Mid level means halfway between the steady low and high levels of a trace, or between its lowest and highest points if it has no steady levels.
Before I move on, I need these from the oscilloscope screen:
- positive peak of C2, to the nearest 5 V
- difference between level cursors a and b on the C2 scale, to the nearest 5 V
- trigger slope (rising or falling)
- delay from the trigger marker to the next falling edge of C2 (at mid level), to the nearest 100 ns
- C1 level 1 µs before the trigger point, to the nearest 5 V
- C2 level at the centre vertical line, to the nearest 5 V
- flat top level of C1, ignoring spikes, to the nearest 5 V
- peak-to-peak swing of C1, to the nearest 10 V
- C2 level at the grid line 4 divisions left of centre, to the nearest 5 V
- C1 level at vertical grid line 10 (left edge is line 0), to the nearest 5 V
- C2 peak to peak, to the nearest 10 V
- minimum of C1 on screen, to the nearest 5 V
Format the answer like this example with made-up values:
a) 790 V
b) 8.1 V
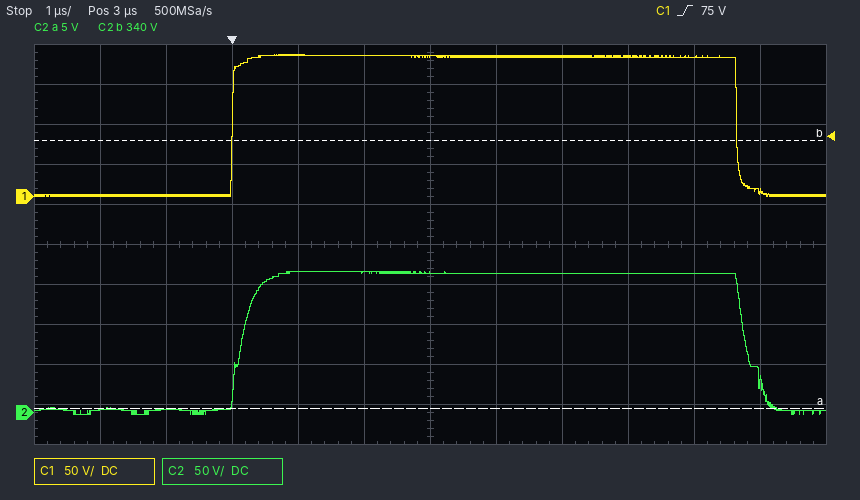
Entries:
a) 175 V
b) 335 V
c) rising
d) 7.8 µs
e) 0 V
f) 175 V
g) 175 V
h) 180 V
i) 5 V
j) 175 V
k) 180 V
l) 0 V
